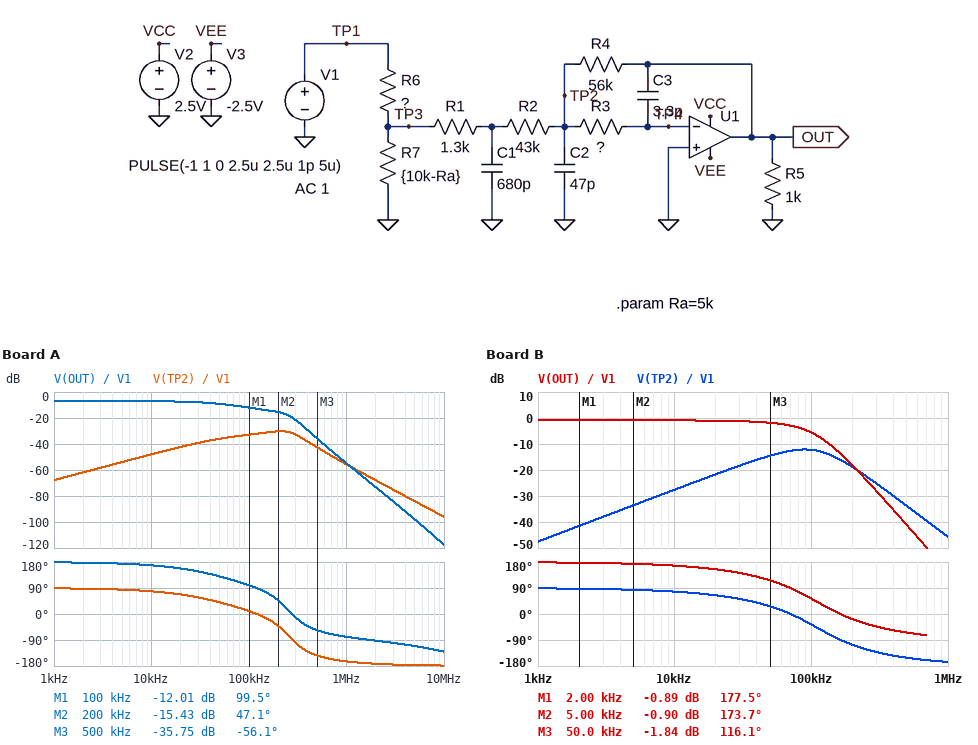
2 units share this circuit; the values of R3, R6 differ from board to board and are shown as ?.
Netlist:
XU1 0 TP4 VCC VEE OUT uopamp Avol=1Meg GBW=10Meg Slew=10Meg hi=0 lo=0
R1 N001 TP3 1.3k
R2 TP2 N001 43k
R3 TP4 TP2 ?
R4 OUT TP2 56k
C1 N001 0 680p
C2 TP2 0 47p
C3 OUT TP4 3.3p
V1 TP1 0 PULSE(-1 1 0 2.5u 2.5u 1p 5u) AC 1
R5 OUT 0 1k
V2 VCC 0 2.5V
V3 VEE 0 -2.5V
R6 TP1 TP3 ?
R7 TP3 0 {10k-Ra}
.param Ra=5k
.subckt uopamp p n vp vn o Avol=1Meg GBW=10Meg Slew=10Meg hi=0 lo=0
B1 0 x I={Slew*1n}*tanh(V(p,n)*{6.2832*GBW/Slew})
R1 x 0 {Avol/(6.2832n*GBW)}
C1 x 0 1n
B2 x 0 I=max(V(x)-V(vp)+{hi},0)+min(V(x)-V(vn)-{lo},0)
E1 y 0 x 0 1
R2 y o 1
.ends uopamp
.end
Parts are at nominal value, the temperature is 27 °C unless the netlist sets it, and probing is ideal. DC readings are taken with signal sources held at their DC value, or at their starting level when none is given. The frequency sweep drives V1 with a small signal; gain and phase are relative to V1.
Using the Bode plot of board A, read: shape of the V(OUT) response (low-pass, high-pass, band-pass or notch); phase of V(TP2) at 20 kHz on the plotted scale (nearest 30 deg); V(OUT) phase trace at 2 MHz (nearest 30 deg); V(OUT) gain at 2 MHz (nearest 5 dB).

low-pass
60 deg
-90 deg
-75 dB
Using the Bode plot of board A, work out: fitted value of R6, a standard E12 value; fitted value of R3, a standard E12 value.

8.2 kΩ
39 kΩ
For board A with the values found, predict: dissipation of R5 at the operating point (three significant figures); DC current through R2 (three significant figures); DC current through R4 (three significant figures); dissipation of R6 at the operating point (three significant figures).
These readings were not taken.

200 µW
7.99 µA
7.99 µA
50.9 µW
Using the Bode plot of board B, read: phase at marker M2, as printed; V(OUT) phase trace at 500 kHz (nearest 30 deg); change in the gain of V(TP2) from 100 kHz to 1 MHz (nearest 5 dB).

173.7 deg
-60 deg
-35 dB
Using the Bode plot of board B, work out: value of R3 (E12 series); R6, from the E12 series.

220 kΩ
1.8 kΩ
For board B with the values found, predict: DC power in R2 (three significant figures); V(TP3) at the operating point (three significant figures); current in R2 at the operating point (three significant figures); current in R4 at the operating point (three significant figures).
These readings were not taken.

11.2 µW
-714 mV
16.1 µA
16.1 µA
